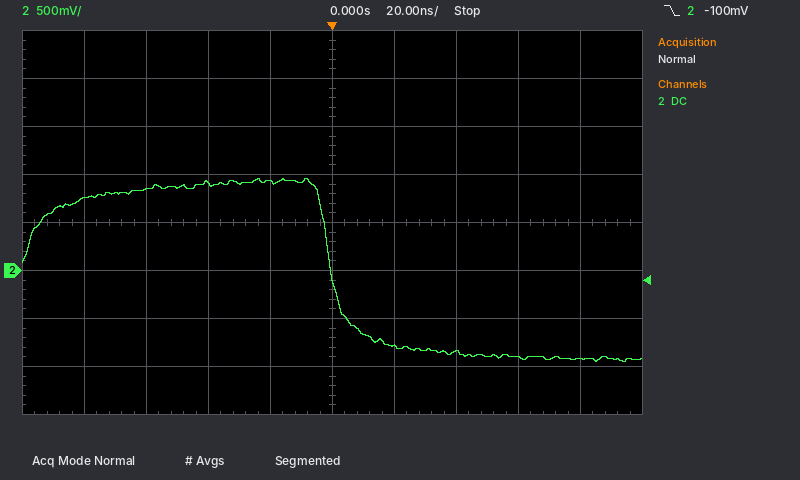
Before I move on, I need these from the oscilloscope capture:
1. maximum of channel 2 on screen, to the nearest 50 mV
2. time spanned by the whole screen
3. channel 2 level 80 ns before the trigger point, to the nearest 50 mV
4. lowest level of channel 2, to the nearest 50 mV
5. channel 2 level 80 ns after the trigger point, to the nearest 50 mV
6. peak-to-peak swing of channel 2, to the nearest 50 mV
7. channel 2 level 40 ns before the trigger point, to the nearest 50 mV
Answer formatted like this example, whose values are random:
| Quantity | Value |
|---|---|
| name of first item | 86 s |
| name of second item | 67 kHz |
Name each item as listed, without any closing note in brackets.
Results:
| Quantity | Value |
|---|---|
| maximum of channel 2 on screen, to the nearest 50 mV | 950 mV |
| time spanned by the whole screen | 200 ns |
| channel 2 level 80 ns before the trigger point, to the nearest 50 mV | 750 mV |
| lowest level of channel 2, to the nearest 50 mV | -950 mV |
| channel 2 level 80 ns after the trigger point, to the nearest 50 mV | -900 mV |
| peak-to-peak swing of channel 2, to the nearest 50 mV | 1.90 V |
| channel 2 level 40 ns before the trigger point, to the nearest 50 mV | 900 mV |
